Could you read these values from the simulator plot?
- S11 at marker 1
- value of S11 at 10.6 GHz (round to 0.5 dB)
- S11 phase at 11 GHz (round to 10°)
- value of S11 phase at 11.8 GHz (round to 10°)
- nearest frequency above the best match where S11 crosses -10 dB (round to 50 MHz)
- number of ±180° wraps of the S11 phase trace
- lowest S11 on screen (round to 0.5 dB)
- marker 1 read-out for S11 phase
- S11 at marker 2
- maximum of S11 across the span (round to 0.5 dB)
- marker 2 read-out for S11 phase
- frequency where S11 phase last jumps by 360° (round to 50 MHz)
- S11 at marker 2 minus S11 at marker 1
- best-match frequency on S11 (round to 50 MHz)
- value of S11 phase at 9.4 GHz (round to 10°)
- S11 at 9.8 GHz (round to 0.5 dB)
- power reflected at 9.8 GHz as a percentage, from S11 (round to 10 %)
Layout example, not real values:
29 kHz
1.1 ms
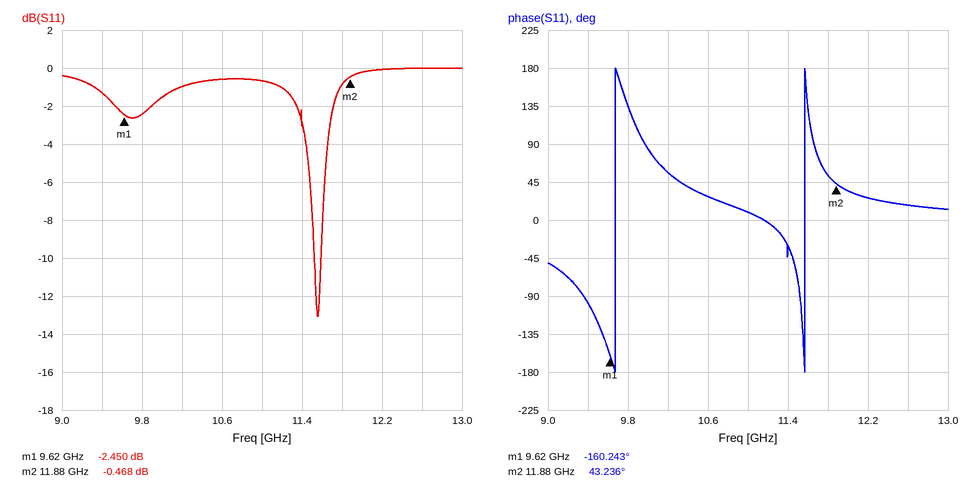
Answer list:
-2.450 dB
-0.5 dB
10°
50°
11.60 GHz
2
-13.0 dB
-160.243°
-0.468 dB
0.0 dB
43.236°
11.55 GHz
1.982 dB
11.55 GHz
-100°
-2.5 dB
60 %
